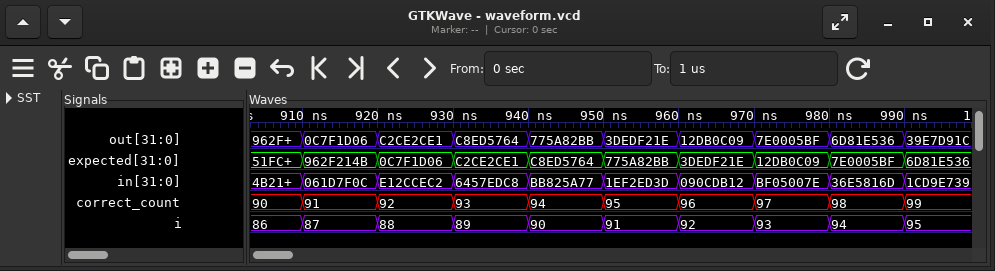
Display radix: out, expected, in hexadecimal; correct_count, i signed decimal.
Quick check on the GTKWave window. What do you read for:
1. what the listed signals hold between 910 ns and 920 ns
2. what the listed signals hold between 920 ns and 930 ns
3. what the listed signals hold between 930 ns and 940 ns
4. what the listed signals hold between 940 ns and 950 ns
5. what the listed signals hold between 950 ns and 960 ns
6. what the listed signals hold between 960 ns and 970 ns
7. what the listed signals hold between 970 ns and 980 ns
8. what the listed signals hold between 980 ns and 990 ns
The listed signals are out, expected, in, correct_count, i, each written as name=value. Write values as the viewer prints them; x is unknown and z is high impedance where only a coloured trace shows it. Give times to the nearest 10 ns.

out=0C7F1D06, expected=962F214B, in=061D7F0C, correct_count=91, i=87
out=C2CE2CE1, expected=0C7F1D06, in=E12CCEC2, correct_count=92, i=88
out=C8ED5764, expected=C2CE2CE1, in=6457EDC8, correct_count=93, i=89
out=775A82BB, expected=C8ED5764, in=BB825A77, correct_count=94, i=90
out=3DEDF21E, expected=775A82BB, in=1EF2ED3D, correct_count=95, i=91
out=12DB0C09, expected=3DEDF21E, in=090CDB12, correct_count=96, i=92
out=7E0005BF, expected=12DB0C09, in=BF05007E, correct_count=97, i=93
out=6D81E536, expected=7E0005BF, in=36E5816D, correct_count=98, i=94
